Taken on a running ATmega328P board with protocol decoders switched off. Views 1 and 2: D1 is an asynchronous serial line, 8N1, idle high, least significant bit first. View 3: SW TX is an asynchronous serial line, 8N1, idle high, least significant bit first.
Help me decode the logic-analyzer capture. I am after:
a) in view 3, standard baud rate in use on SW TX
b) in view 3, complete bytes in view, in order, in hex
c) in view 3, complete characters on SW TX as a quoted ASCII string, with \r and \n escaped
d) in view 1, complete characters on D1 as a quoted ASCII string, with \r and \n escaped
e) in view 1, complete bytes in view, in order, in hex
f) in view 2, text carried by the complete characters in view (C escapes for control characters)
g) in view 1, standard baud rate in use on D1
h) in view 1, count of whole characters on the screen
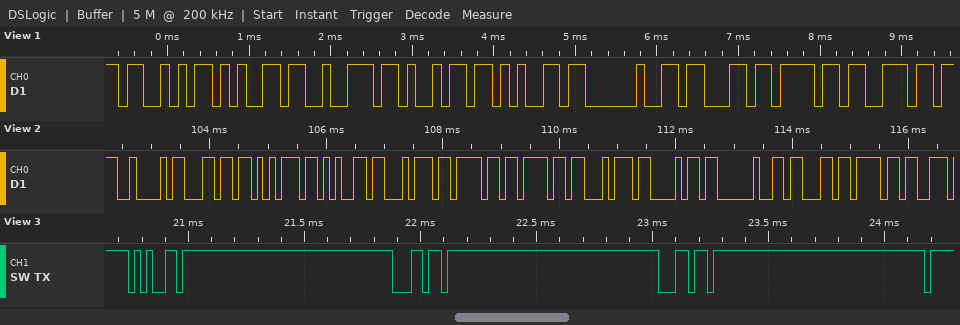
38400 baud
65 6C 6C
"ell"
"Serie con"
0x53 0x65 0x72 0x69 0x65 0x20 0x63 0x6F 0x6E
"Bluetooth co"
9600 baud
9
